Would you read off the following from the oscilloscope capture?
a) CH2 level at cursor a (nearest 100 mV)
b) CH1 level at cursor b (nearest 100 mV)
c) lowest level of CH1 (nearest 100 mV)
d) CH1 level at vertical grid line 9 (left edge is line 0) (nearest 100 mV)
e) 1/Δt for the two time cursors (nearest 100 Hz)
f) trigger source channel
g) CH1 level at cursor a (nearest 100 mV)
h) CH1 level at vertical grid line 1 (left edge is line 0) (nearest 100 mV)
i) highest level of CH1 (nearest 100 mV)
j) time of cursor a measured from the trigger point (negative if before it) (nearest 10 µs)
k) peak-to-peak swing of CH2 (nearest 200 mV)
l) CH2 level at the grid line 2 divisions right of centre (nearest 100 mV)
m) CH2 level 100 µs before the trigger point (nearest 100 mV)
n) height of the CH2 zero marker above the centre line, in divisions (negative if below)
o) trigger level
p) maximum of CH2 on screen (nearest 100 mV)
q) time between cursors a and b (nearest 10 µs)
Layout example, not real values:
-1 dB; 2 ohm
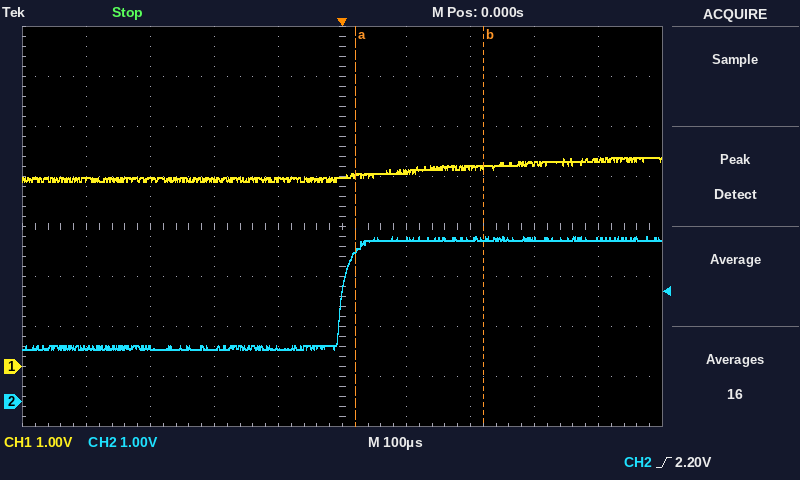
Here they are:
3.0 V; 4.0 V; 3.7 V; 4.1 V; 5.0 kHz; CH2; 3.8 V; 3.7 V; 4.2 V; +20 µs; 2.2 V; 3.2 V; 1.1 V; -3.5 div; 2.20 V; 3.3 V; 200 µs
